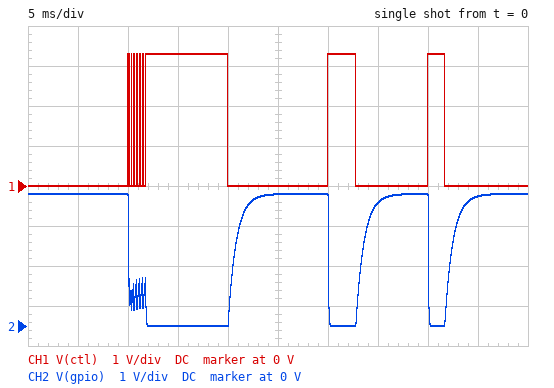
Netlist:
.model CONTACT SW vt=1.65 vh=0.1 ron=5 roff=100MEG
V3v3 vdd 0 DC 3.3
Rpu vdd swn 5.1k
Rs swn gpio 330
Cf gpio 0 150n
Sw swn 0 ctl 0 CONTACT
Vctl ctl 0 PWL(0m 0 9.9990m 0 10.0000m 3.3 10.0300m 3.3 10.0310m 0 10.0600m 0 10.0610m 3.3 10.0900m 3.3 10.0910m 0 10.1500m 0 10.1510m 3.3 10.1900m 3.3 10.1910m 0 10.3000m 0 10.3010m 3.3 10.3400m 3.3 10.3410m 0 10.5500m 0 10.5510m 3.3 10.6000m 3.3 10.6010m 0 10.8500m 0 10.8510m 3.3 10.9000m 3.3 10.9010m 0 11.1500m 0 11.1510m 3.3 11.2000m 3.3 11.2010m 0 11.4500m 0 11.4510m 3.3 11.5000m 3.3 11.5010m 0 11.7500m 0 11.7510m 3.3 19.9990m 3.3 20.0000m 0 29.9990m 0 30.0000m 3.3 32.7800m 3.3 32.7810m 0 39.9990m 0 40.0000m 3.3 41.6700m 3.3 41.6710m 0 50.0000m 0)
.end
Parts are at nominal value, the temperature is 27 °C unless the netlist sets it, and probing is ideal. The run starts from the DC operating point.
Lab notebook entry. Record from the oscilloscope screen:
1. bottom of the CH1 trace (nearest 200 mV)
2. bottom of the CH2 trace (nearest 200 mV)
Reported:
0 V
0 V
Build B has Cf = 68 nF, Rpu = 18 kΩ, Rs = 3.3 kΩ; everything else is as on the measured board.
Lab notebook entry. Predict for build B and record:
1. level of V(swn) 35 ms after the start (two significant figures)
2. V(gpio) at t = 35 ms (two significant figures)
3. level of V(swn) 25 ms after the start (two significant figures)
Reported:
2.7 V
2.6 V
3.2 V
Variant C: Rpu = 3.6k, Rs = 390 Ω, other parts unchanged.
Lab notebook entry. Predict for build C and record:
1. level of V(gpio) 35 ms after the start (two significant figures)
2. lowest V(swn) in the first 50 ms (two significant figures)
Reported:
3.2 V
4.6 mV
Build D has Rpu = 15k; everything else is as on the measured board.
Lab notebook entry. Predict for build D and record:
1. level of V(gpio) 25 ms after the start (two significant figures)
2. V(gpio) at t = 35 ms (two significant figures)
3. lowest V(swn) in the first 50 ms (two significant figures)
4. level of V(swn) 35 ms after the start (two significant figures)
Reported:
2.9 V
2.0 V
1.1 mV
2.1 V
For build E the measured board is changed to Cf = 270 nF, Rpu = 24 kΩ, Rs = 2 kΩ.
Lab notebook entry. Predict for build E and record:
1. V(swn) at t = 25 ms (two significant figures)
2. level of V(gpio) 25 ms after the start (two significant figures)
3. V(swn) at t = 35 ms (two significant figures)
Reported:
1.8 V
1.7 V
1.1 V
